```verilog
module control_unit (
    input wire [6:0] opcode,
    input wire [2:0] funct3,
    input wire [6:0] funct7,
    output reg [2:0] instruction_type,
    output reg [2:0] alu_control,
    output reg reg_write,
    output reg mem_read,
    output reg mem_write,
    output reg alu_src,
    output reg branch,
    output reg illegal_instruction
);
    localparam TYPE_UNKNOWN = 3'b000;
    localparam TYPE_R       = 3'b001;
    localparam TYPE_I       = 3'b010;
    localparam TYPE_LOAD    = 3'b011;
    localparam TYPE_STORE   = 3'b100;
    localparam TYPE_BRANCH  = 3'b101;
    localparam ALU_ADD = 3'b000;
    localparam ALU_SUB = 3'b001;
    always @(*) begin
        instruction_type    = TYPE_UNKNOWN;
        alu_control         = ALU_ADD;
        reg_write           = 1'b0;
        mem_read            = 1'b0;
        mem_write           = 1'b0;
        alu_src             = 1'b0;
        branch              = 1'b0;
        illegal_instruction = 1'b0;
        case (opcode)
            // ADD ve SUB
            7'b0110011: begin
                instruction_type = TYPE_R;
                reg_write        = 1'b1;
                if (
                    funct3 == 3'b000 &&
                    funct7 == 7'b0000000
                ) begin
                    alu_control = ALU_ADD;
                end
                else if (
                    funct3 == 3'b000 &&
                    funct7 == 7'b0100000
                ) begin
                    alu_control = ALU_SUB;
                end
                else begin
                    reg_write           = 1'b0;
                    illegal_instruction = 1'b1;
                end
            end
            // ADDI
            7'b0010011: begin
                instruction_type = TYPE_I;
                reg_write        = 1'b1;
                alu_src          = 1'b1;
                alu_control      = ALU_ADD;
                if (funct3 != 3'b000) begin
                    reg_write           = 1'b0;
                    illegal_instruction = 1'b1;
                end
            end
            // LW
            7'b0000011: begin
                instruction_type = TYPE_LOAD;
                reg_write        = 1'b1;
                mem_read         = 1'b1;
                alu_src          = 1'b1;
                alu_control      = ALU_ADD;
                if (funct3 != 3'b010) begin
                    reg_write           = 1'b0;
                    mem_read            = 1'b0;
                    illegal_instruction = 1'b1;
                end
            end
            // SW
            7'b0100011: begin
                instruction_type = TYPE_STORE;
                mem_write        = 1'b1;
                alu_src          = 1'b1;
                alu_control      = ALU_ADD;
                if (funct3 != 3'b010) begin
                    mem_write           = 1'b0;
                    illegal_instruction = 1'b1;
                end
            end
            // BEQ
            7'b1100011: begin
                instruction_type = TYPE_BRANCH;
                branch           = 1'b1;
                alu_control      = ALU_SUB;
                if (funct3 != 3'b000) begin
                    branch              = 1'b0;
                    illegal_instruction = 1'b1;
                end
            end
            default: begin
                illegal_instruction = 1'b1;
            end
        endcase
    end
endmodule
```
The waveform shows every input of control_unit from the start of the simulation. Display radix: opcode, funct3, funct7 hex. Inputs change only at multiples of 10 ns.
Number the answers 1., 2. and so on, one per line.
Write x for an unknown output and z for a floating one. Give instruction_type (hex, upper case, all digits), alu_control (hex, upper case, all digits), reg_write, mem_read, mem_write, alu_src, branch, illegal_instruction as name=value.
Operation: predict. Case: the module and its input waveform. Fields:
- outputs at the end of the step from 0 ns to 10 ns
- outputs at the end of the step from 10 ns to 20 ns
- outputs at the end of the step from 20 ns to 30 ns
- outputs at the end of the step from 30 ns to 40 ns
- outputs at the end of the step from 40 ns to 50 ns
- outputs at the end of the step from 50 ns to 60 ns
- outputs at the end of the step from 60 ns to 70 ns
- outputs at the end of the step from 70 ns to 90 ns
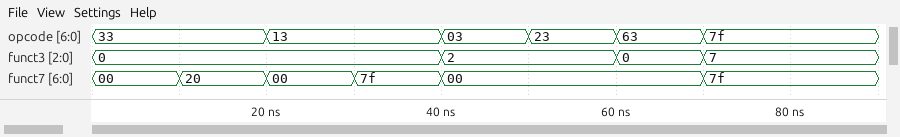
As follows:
1. instruction_type=1, alu_control=0, reg_write=1, mem_read=0, mem_write=0, alu_src=0, branch=0, illegal_instruction=0
2. instruction_type=1, alu_control=1, reg_write=1, mem_read=0, mem_write=0, alu_src=0, branch=0, illegal_instruction=0
3. instruction_type=2, alu_control=0, reg_write=1, mem_read=0, mem_write=0, alu_src=1, branch=0, illegal_instruction=0
4. instruction_type=2, alu_control=0, reg_write=1, mem_read=0, mem_write=0, alu_src=1, branch=0, illegal_instruction=0
5. instruction_type=3, alu_control=0, reg_write=1, mem_read=1, mem_write=0, alu_src=1, branch=0, illegal_instruction=0
6. instruction_type=4, alu_control=0, reg_write=0, mem_read=0, mem_write=1, alu_src=1, branch=0, illegal_instruction=0
7. instruction_type=5, alu_control=1, reg_write=0, mem_read=0, mem_write=0, alu_src=0, branch=1, illegal_instruction=0
8. instruction_type=0, alu_control=0, reg_write=0, mem_read=0, mem_write=0, alu_src=0, branch=0, illegal_instruction=1
